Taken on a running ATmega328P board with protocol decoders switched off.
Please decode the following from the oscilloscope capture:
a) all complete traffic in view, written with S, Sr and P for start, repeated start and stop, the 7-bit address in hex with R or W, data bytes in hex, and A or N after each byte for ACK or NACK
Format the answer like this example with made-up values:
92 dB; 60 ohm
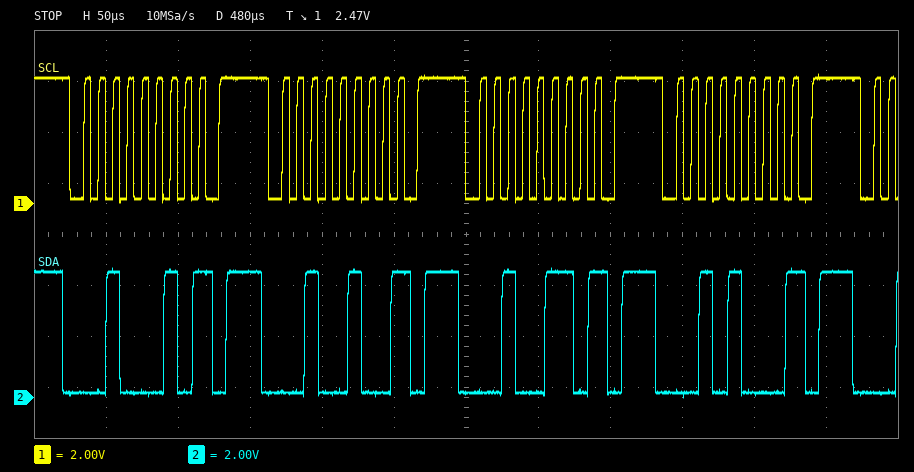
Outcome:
S 11W N P S 12W N P S 13W N P S 14W N P
